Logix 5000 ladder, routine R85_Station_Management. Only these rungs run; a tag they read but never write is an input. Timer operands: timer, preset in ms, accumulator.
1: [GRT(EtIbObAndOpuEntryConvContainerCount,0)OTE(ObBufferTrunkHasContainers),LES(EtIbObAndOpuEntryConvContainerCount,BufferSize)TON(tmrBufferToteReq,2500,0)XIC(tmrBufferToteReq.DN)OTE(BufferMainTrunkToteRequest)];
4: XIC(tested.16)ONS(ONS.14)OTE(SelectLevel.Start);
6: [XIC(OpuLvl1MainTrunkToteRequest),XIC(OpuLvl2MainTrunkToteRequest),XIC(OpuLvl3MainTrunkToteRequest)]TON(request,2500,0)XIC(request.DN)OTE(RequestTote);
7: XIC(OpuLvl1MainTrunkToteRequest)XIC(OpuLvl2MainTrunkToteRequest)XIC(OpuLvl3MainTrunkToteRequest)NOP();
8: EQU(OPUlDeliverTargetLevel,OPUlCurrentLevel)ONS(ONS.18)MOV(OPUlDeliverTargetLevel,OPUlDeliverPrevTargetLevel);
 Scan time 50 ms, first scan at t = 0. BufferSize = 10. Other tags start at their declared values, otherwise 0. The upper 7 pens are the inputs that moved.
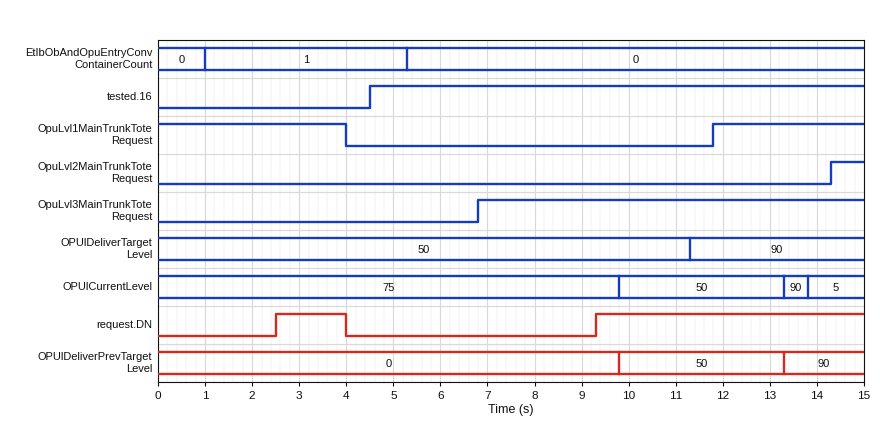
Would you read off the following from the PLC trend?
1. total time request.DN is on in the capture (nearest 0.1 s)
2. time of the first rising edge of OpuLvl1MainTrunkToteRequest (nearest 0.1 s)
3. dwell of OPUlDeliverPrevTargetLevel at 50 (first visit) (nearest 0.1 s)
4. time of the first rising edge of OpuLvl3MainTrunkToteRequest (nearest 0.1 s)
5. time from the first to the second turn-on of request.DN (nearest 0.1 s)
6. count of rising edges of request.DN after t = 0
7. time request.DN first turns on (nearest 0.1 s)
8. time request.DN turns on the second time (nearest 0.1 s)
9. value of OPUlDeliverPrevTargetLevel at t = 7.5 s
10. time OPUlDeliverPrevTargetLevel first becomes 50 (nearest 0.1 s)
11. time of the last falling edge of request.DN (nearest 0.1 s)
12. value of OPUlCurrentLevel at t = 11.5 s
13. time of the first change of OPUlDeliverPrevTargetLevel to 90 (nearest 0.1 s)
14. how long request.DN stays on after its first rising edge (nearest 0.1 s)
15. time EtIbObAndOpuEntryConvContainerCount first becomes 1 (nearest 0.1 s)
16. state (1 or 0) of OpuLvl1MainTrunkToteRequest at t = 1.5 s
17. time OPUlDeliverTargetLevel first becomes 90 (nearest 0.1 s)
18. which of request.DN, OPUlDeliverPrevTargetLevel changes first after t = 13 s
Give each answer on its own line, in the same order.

7.2 s
11.8 s
3.5 s
6.8 s
6.8 s
2
2.5 s
9.3 s
0
9.8 s
4.0 s
50
13.3 s
1.5 s
1.0 s
1
11.3 s
OPUlDeliverPrevTargetLevel
